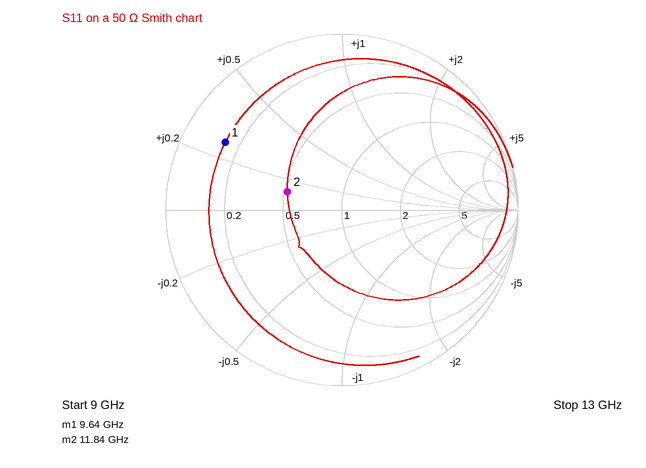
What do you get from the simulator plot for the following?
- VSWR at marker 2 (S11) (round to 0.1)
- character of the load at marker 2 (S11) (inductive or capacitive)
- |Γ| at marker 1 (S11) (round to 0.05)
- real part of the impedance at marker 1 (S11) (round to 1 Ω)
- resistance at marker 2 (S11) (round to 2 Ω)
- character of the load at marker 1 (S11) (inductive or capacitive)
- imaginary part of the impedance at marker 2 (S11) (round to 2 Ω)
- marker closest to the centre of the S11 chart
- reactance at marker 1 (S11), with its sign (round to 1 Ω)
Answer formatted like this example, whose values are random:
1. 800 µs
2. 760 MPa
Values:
1. 2.0
2. inductive
3. 0.75
4. 7 Ω
5. 26 Ω
6. inductive
7. +6 Ω
8. marker 2
9. +13 Ω
